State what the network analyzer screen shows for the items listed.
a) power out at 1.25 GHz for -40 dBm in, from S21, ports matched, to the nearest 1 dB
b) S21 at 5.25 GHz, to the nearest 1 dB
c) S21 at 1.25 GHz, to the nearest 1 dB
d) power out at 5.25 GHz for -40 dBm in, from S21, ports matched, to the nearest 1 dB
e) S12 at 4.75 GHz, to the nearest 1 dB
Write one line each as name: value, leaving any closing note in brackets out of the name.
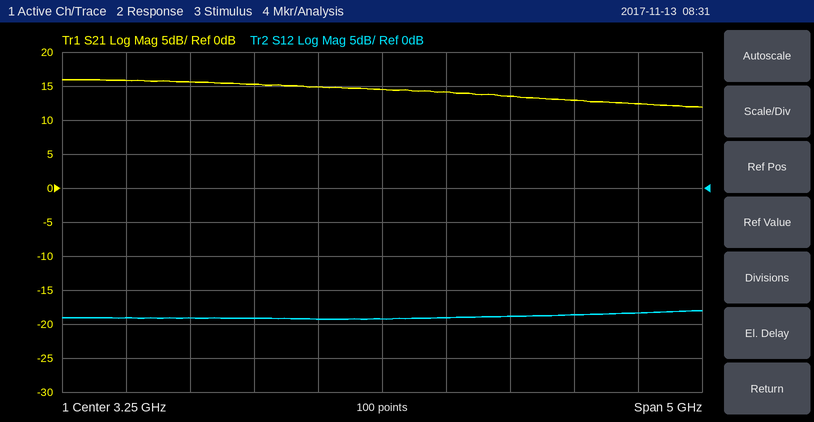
power out at 1.25 GHz for -40 dBm in, from S21, ports matched, to the nearest 1 dB: -24 dBm
S21 at 5.25 GHz, to the nearest 1 dB: 12 dB
S21 at 1.25 GHz, to the nearest 1 dB: 16 dB
power out at 5.25 GHz for -40 dBm in, from S21, ports matched, to the nearest 1 dB: -28 dBm
S12 at 4.75 GHz, to the nearest 1 dB: -19 dB
